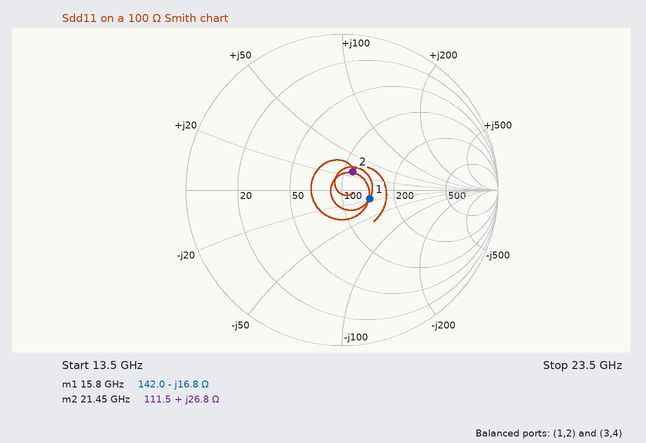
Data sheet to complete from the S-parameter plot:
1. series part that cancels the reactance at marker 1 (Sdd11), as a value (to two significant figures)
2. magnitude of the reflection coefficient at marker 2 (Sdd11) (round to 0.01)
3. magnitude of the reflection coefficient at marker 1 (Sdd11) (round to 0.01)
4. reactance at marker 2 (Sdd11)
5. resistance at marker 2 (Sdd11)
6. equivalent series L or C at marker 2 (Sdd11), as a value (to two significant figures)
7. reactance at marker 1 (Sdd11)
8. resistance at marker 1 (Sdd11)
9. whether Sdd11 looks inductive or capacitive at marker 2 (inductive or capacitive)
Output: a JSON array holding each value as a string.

["170 pH", "0.14", "0.19", "+26.8 Ω", "111.5 Ω", "200 pH", "-16.8 Ω", "142.0 Ω", "inductive"]
